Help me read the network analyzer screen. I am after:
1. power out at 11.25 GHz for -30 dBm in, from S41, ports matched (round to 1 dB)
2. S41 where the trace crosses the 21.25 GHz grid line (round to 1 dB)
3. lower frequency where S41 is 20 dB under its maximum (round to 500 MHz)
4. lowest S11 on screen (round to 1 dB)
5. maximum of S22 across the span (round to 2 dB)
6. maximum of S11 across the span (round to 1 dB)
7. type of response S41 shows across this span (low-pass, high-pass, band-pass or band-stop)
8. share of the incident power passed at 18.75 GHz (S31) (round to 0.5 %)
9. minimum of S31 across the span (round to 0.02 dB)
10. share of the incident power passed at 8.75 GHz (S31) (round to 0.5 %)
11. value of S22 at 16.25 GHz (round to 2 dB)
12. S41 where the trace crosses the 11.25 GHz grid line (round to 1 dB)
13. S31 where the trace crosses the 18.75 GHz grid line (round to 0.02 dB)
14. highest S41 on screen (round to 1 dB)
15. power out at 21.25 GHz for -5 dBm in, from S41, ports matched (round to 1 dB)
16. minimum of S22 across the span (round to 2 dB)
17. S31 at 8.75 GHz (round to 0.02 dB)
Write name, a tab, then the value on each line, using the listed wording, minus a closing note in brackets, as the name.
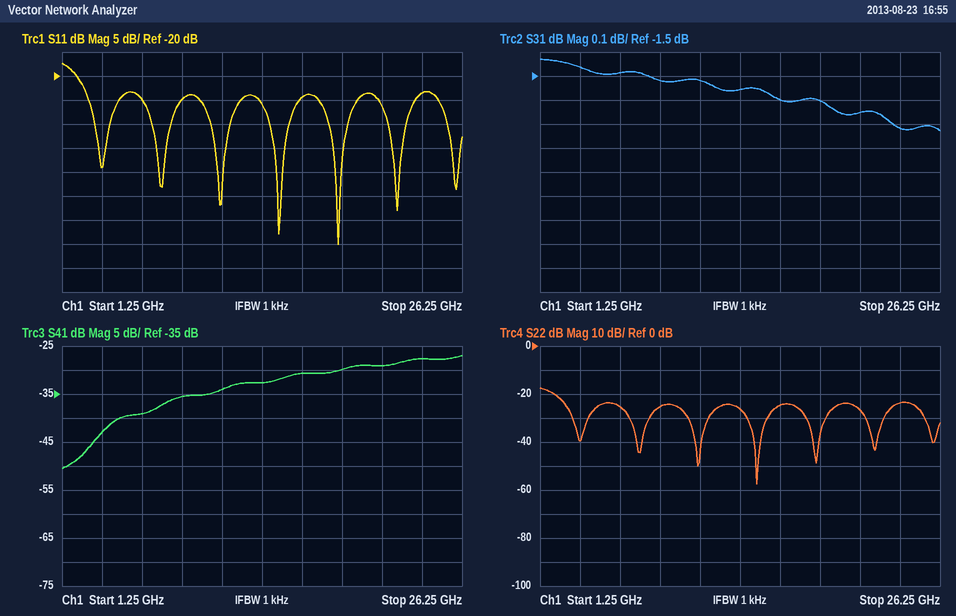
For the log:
power out at 11.25 GHz for -30 dBm in, from S41, ports matched	-64 dBm
S41 where the trace crosses the 21.25 GHz grid line	-29 dB
lower frequency where S41 is 20 dB under its maximum	2.5 GHz
lowest S11 on screen	-55 dB
maximum of S22 across the span	-18 dB
maximum of S11 across the span	-17 dB
type of response S41 shows across this span	high-pass
share of the incident power passed at 18.75 GHz (S31)	69.0 %
minimum of S31 across the span	-1.72 dB
share of the incident power passed at 8.75 GHz (S31)	70.5 %
value of S22 at 16.25 GHz	-24 dB
S41 where the trace crosses the 11.25 GHz grid line	-34 dB
S31 where the trace crosses the 18.75 GHz grid line	-1.60 dB
highest S41 on screen	-27 dB
power out at 21.25 GHz for -5 dBm in, from S41, ports matched	-34 dBm
minimum of S22 across the span	-58 dB
S31 at 8.75 GHz	-1.52 dB
